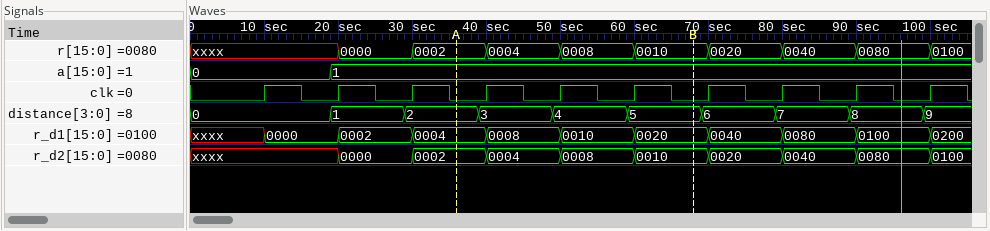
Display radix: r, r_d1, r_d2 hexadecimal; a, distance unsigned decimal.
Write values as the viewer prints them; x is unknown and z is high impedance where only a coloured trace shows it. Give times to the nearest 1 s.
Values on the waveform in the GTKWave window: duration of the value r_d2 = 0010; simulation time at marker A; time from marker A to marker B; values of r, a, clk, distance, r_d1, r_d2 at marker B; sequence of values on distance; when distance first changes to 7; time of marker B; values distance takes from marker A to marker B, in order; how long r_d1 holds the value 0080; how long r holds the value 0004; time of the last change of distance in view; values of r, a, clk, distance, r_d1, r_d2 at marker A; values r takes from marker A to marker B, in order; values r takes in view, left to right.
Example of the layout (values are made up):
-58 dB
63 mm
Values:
10 s
36 s
32 s
r=0010, a=1, clk=0, distance=5, r_d1=0020, r_d2=0010
0, 1, 2, 3, 4, 5, 6, 7, 8, 9
79 s
68 s
2, 3, 4, 5
10 s
10 s
99 s
r=0002, a=1, clk=0, distance=2, r_d1=0004, r_d2=0002
0002, 0004, 0008, 0010
xxxx, 0000, 0002, 0004, 0008, 0010, 0020, 0040, 0080, 0100
